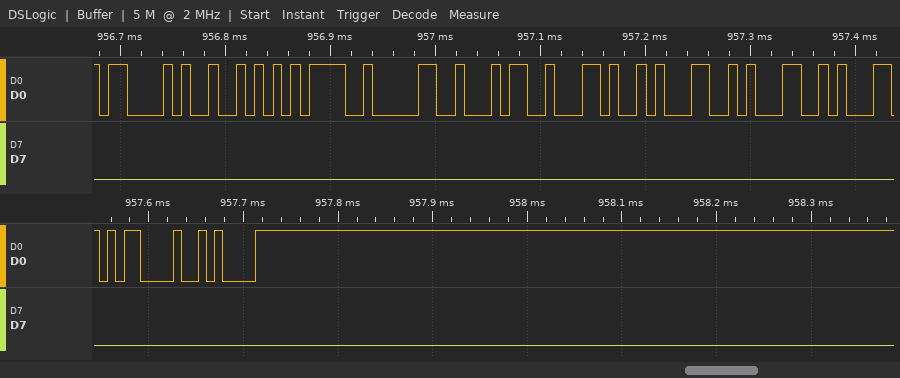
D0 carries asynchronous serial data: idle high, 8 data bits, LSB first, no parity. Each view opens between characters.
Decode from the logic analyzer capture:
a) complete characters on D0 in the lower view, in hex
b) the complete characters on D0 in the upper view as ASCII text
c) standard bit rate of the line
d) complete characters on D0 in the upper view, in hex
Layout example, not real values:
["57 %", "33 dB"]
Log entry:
["0D, 0A", "\"CR=04,11\"", "115200 baud", "43, 52, 3D, 30, 34, 2C, 31, 31"]
